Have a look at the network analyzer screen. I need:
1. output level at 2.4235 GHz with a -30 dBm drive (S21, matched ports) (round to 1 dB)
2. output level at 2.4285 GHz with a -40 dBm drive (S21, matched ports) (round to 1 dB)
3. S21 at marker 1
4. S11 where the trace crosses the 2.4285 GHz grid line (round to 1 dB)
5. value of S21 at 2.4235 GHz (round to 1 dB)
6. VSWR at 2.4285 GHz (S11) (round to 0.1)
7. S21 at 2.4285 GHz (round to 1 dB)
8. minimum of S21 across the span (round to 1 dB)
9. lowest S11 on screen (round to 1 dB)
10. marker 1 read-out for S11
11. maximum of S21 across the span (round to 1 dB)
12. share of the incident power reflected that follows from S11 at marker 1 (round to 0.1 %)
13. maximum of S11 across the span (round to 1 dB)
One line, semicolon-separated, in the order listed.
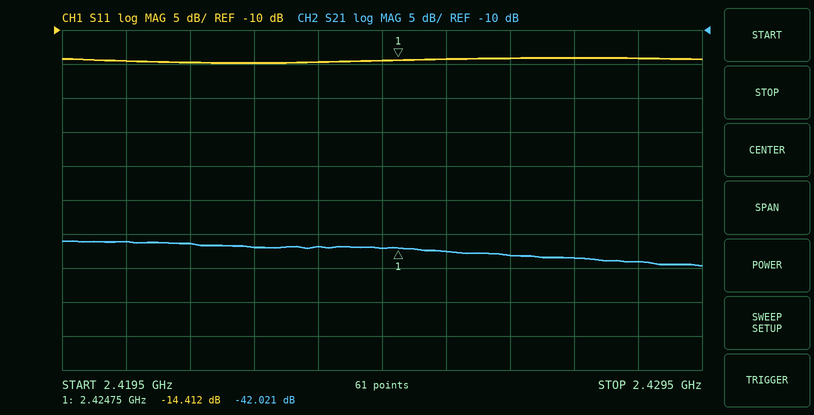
-72 dBm; -84 dBm; -42.021 dB; -14 dB; -42 dB; 1.5; -44 dB; -45 dB; -15 dB; -14.412 dB; -41 dB; 3.6 %; -14 dB
